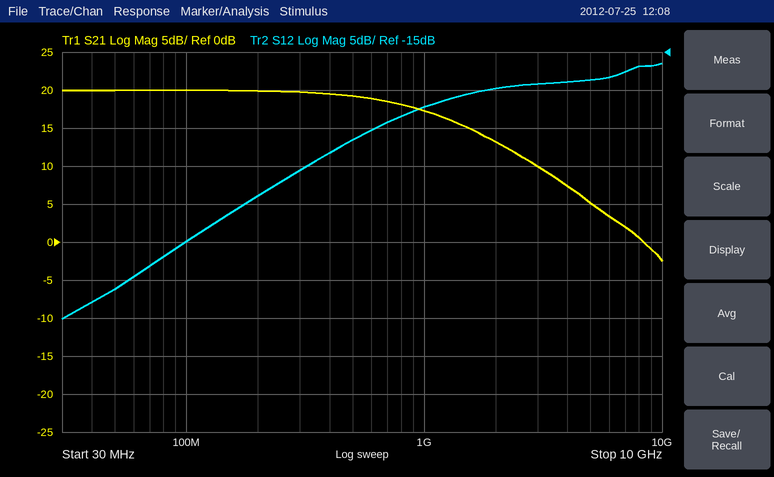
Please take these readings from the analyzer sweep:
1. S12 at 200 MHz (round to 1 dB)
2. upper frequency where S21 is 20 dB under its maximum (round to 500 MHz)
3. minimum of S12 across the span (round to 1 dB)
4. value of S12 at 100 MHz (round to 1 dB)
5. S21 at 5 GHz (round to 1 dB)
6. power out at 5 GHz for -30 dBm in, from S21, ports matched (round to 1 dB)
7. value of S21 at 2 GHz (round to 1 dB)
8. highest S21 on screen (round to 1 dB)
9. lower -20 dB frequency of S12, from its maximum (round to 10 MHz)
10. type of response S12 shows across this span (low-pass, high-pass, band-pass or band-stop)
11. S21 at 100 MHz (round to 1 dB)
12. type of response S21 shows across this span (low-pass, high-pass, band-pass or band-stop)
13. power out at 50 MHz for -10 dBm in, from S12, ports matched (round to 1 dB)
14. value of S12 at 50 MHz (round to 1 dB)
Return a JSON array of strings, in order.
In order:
["-34 dB", "8.5 GHz", "-50 dB", "-40 dB", "5 dB", "-25 dBm", "13 dB", "20 dB", "150 MHz", "high-pass", "20 dB", "low-pass", "-56 dBm", "-46 dB"]
